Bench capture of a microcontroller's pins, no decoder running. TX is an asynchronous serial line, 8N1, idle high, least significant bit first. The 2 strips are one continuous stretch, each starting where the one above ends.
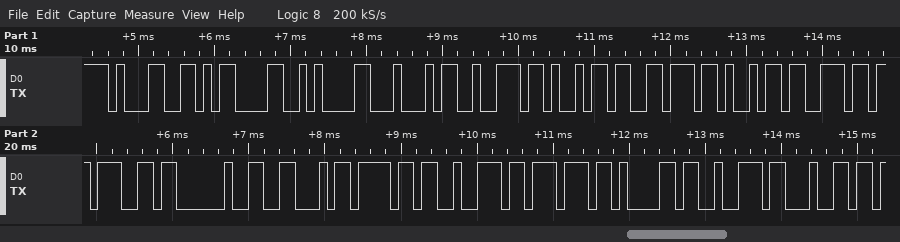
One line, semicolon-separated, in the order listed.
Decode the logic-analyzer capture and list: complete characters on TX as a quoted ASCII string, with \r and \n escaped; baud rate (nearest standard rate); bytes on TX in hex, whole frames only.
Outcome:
"1\r\nDriving Forward"; 9600 baud; 31 0D 0A 44 72 69 76 69 6E 67 20 46 6F 72 77 61 72 64
